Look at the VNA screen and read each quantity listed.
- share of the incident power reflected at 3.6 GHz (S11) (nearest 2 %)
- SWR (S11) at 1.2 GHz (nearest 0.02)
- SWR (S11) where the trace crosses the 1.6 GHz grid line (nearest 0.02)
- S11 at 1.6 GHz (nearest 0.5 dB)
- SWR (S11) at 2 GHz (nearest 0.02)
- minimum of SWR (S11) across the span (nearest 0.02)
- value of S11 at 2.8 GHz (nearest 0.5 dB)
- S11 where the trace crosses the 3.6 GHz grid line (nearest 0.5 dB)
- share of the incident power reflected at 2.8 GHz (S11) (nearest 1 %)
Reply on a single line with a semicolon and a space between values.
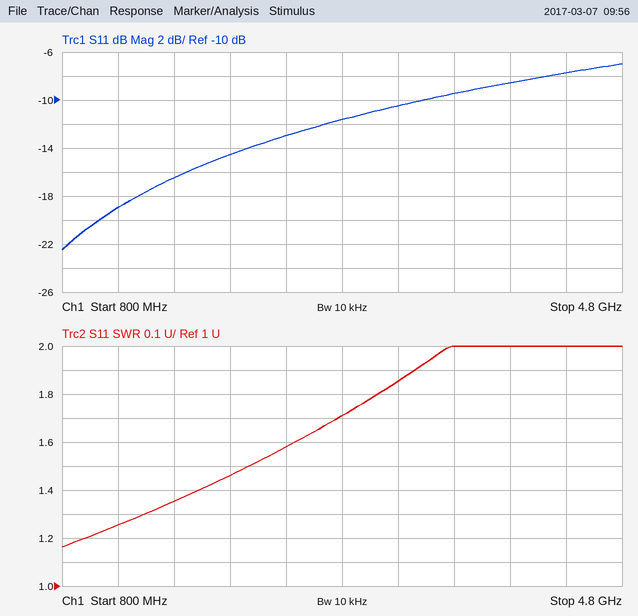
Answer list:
12 %; 1.26; 1.36; -16.5 dB; 1.46; 1.16; -11.5 dB; -9.5 dB; 7 %
